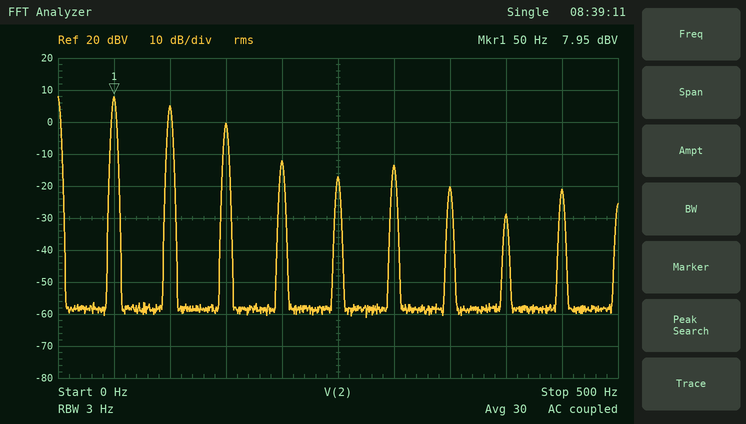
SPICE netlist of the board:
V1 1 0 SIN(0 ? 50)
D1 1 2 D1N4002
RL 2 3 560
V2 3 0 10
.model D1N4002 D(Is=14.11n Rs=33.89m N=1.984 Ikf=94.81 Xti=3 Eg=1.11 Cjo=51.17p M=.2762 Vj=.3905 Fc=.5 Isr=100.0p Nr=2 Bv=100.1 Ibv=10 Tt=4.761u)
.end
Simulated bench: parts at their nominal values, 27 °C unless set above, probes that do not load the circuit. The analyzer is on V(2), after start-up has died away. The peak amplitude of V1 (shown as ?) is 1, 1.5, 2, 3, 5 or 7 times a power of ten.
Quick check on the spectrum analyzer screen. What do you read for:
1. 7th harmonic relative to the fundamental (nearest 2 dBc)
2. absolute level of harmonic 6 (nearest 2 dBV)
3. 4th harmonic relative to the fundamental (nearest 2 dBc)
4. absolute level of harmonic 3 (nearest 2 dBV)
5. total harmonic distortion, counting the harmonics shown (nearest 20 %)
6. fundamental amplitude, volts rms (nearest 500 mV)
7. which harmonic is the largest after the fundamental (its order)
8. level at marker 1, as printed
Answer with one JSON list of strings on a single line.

["-28 dBc", "-14 dBV", "-20 dBc", "0 dBV", "80 %", "2.5 V", "2", "7.95 dBV"]
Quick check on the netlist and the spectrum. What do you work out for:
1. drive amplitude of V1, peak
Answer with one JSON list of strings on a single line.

["20 V"]
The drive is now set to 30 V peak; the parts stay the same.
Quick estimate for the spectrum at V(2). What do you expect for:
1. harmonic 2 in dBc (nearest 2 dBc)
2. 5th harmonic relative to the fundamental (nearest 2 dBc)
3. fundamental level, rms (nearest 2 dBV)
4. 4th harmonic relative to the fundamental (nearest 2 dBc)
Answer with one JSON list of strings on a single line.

["-4 dBc", "-22 dBc", "16 dBV", "-30 dBc"]
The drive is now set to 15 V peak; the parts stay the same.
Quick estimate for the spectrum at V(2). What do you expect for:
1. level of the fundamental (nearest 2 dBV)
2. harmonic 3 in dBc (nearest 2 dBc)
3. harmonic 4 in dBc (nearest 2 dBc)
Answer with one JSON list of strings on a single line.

["0 dBV", "-4 dBc", "-10 dBc"]
